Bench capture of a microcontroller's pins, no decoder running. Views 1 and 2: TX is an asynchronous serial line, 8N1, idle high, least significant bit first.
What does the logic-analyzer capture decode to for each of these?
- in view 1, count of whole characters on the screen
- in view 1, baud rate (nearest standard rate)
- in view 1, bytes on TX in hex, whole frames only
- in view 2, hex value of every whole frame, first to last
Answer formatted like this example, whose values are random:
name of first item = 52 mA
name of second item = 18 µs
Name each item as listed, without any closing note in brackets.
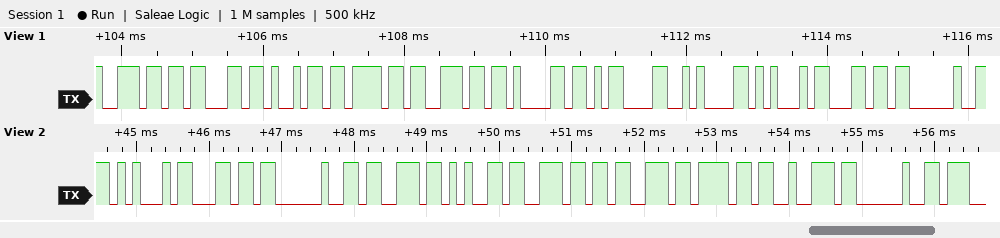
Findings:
in view 1, count of whole characters on the screen = 11
in view 1, baud rate = 9600 baud
in view 1, bytes on TX in hex, whole frames only = 6E 63 69 6F 6E 61 0D 0A 45 6C 20
in view 2, hex value of every whole frame, first to last = 0x45 0x6C 0x20 0x73 0x65 0x6E 0x73 0x6F 0x72 0x20
